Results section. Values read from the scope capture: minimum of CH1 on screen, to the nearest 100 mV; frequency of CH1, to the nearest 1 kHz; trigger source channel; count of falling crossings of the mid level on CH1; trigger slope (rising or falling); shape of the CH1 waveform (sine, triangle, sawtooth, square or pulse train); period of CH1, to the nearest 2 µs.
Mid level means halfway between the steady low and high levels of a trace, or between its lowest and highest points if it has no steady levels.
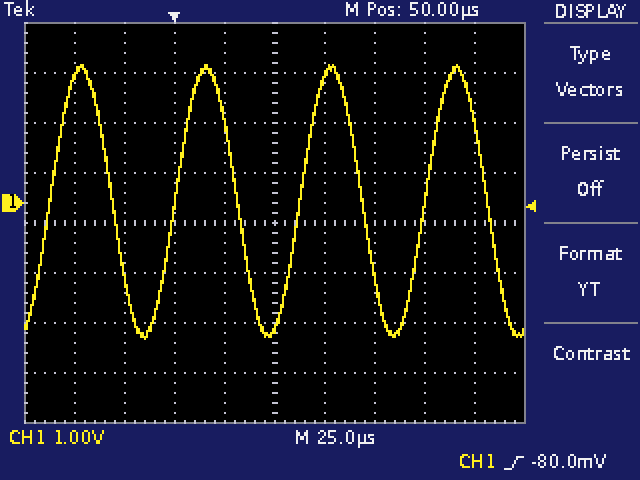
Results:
-2.7 V
16 kHz
CH1
4
rising
sine
62 µs
